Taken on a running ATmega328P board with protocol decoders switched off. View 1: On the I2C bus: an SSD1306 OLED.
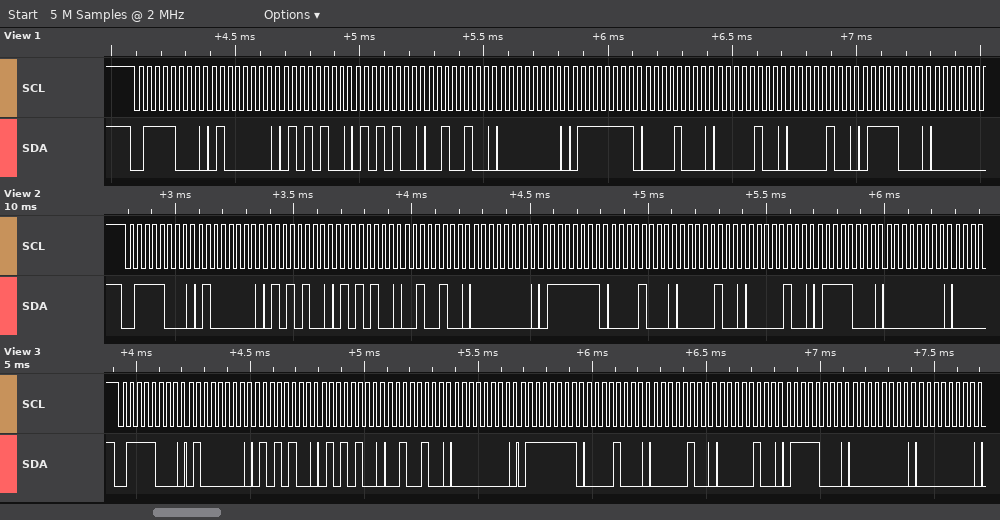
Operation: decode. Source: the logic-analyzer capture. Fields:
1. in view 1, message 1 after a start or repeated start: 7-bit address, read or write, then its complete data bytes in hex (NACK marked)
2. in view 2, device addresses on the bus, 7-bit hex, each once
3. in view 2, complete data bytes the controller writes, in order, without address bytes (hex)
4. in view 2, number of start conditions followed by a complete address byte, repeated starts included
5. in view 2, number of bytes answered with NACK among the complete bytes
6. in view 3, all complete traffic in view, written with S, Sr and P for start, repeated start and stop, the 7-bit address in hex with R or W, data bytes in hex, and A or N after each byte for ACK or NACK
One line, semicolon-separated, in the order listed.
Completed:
0x3C write: 40 54 54 24 00 7F 08 04 04 78; 0x3C; 40 54 54 24 00 7F 08 04 04 78 00; 1; 0; S 3CW A 40 A 54 A 54 A 24 A 00 A 7F A 08 A 04 A 04 A 78 A 00 A 00 A
